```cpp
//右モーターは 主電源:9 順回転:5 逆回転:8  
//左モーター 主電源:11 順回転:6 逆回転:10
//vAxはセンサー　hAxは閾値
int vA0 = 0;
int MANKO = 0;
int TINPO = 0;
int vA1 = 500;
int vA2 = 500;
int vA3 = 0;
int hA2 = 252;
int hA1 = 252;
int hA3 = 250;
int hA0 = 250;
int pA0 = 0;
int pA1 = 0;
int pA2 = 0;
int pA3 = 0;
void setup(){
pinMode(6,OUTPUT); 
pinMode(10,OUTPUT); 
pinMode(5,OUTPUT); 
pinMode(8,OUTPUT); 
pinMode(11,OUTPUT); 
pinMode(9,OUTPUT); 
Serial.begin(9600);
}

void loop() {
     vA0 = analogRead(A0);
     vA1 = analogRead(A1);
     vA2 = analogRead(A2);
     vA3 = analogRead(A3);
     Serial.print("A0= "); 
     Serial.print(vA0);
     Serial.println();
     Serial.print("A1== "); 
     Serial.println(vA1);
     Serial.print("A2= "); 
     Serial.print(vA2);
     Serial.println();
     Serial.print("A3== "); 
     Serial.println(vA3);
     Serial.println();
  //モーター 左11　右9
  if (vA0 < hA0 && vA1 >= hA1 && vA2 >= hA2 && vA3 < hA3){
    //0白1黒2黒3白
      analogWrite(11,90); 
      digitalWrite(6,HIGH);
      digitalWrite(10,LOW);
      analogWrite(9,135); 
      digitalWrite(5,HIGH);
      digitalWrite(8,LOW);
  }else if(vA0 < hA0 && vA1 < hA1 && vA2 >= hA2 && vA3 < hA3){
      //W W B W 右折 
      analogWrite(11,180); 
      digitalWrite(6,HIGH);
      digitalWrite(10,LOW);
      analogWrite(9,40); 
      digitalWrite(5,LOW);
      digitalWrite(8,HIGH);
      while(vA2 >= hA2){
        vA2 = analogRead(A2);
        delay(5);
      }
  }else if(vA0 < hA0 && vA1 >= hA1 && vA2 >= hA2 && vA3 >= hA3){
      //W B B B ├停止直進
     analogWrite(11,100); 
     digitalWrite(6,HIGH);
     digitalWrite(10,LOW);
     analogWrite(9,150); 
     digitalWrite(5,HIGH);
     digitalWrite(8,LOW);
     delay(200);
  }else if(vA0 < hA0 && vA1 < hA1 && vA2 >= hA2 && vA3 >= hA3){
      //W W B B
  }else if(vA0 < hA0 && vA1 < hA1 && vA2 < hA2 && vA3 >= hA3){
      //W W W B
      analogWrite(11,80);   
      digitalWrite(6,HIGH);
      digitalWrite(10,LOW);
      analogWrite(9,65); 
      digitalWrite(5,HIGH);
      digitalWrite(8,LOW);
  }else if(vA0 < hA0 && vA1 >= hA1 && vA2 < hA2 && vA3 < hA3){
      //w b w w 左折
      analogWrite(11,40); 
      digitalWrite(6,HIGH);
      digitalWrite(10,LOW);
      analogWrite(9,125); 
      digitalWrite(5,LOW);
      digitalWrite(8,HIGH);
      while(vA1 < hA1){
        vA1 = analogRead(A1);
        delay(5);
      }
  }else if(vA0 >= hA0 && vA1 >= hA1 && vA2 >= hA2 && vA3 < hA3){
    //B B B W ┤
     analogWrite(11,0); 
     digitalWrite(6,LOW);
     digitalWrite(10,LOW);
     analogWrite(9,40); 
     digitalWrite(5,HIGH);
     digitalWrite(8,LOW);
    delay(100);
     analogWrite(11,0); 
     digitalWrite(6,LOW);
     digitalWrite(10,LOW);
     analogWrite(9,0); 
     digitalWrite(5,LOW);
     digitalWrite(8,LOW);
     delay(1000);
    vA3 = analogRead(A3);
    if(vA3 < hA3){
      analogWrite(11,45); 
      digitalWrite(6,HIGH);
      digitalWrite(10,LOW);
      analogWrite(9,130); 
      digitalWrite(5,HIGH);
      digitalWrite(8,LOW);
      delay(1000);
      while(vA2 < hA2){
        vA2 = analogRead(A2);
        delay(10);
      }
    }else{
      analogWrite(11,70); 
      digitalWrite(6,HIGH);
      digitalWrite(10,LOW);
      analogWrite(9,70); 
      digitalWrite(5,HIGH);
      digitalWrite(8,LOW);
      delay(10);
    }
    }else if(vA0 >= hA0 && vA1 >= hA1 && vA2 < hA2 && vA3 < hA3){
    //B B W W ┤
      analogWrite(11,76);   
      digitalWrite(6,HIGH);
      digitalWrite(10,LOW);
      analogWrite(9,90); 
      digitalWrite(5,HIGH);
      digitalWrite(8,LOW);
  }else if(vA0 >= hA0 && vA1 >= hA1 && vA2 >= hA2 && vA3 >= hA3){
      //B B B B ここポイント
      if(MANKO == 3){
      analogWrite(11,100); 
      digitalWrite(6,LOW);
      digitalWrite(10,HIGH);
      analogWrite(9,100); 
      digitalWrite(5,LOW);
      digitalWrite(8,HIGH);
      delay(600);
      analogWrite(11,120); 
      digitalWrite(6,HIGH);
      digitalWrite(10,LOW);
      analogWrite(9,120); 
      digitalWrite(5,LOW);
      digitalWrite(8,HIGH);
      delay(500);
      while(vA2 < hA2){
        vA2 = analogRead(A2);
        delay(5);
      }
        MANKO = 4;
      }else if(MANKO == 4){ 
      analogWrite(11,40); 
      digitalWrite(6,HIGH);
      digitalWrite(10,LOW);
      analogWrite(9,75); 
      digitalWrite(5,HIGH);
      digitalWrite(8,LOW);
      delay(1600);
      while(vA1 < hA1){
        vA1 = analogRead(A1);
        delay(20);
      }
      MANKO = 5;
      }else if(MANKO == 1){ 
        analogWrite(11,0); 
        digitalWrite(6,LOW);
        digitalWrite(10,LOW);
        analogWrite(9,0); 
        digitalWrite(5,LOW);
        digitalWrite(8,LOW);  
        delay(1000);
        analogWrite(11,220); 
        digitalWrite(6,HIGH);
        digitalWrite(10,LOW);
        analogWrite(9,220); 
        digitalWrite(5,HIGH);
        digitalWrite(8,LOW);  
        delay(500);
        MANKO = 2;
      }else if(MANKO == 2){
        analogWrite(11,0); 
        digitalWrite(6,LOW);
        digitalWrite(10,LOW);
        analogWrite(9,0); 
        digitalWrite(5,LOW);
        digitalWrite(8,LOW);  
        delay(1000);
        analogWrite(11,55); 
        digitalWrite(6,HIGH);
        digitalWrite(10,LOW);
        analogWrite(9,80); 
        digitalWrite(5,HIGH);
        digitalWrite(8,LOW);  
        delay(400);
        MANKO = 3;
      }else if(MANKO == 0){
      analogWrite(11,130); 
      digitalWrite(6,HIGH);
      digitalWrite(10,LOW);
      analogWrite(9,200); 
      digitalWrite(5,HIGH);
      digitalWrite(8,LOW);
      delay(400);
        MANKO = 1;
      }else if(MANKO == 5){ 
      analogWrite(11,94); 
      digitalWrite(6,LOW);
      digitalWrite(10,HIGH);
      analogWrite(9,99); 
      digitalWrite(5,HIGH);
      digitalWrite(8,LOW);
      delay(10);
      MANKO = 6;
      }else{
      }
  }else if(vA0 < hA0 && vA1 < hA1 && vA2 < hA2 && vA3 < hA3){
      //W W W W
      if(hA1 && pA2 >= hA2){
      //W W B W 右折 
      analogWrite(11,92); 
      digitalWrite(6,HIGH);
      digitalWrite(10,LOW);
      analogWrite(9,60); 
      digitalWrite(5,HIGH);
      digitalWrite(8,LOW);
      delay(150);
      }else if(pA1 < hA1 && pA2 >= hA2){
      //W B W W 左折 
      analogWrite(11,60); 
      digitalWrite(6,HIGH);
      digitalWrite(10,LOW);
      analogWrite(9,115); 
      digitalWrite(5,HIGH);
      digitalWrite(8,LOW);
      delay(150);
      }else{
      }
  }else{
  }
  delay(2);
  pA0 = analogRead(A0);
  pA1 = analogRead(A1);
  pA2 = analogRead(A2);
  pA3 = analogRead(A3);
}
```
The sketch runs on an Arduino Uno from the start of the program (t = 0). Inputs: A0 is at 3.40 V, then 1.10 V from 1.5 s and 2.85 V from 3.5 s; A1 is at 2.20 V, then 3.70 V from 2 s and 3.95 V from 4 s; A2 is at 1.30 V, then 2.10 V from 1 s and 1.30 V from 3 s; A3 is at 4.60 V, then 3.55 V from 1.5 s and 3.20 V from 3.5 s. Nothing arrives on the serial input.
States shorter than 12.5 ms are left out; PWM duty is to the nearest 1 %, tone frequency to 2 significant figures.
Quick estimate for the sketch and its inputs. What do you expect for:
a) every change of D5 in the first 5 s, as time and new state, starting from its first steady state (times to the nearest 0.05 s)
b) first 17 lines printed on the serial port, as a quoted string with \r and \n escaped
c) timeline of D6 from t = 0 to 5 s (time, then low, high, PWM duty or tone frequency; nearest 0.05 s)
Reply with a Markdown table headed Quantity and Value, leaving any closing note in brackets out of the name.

| Quantity | Value |
|---|---|
| every change of D5 in the first 5 s, as time and new state, starting from its first steady state | 0 s high; 0.4 s low; 1.4 s high; 3.55 s low; 4.55 s high; 4.95 s low |
| first 17 lines printed on the serial port, as a quoted string with \r and \n escaped | "A0= 696\r\nA1== 450\r\nA2= 266\r\nA3== 942\r\n\r\nA0= 696\r\nA1== 450\r\nA2= 266\r\nA3== 942\r\n\r\nA0= 225\r\nA1== 450\r\nA2= 430\r\nA3== 727\r\n\r\nA0= 225\r\nA1== 757\r\n" |
| timeline of D6 from t = 0 to 5 s | 0 s high; 0.4 s low; 1.4 s high; 3.55 s low; 4.55 s high; 4.95 s low |
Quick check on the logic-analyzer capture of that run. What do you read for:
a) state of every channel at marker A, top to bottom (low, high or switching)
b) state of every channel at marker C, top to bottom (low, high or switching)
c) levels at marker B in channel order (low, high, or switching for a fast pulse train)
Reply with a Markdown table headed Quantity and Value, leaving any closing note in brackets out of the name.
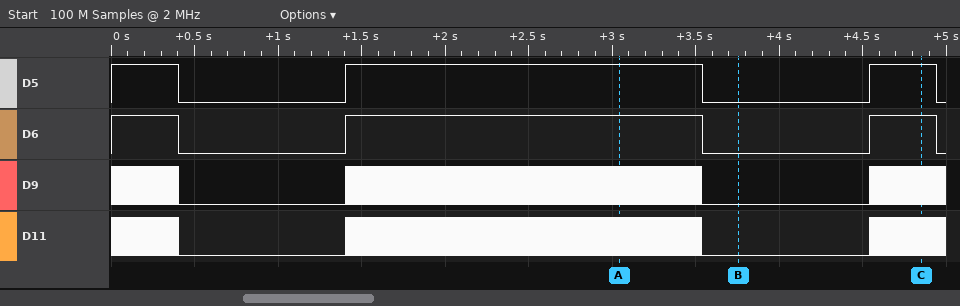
| Quantity | Value |
|---|---|
| state of every channel at marker A, top to bottom | D5 high, D6 high, D9 switching, D11 switching |
| state of every channel at marker C, top to bottom | D5 high, D6 high, D9 switching, D11 switching |
| levels at marker B in channel order | D5 low, D6 low, D9 low, D11 low |
